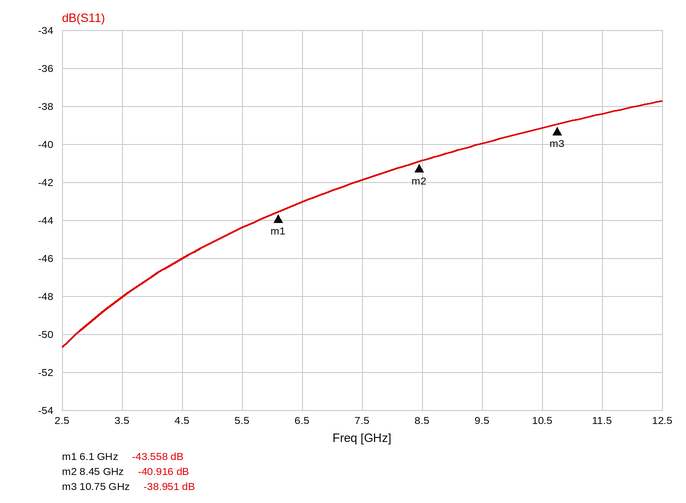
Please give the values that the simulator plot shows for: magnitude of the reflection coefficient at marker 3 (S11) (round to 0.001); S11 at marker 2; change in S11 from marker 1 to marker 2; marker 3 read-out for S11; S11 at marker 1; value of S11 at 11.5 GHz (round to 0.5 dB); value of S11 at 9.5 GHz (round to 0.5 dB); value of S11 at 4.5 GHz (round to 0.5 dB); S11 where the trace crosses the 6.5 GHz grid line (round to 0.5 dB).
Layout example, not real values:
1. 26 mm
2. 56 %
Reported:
1. 0.011
2. -40.916 dB
3. 2.642 dB
4. -38.951 dB
5. -43.558 dB
6. -38.5 dB
7. -40.0 dB
8. -46.0 dB
9. -43.0 dB
